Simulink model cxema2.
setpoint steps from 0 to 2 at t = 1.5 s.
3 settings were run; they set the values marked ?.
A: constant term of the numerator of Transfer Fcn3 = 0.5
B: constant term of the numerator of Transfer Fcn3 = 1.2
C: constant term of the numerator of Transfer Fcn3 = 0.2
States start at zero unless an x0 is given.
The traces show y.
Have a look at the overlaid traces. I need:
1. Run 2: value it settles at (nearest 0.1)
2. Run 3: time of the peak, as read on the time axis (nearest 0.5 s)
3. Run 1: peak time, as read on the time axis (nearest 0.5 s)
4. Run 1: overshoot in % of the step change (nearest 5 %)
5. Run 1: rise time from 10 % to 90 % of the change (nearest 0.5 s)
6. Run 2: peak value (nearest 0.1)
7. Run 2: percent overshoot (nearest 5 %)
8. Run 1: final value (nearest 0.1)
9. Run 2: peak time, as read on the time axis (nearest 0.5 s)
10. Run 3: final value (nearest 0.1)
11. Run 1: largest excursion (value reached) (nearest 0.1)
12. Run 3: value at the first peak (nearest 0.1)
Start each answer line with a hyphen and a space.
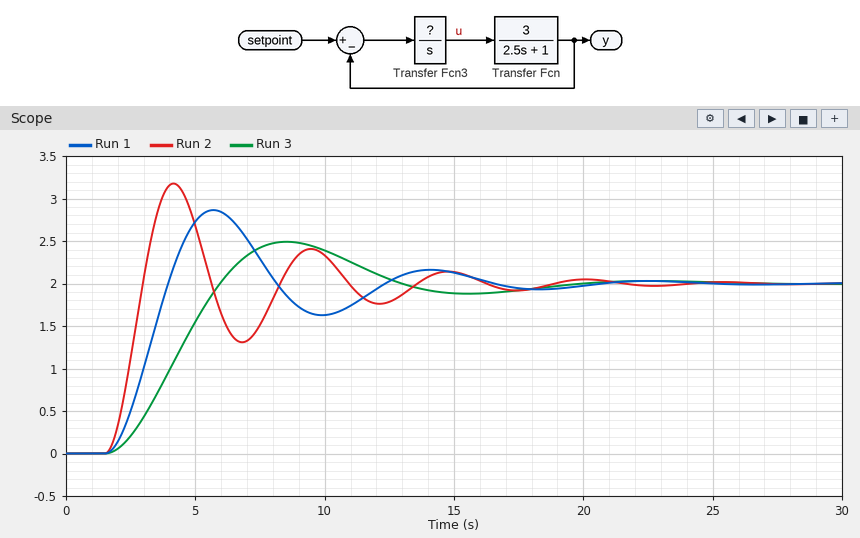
- 2.0
- 8.5 s
- 5.5 s
- 45 %
- 1.5 s
- 3.2
- 60 %
- 2.0
- 4.0 s
- 2.0
- 2.9
- 2.5
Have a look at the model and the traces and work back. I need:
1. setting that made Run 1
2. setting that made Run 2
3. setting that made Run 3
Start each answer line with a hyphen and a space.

- A
- B
- C
